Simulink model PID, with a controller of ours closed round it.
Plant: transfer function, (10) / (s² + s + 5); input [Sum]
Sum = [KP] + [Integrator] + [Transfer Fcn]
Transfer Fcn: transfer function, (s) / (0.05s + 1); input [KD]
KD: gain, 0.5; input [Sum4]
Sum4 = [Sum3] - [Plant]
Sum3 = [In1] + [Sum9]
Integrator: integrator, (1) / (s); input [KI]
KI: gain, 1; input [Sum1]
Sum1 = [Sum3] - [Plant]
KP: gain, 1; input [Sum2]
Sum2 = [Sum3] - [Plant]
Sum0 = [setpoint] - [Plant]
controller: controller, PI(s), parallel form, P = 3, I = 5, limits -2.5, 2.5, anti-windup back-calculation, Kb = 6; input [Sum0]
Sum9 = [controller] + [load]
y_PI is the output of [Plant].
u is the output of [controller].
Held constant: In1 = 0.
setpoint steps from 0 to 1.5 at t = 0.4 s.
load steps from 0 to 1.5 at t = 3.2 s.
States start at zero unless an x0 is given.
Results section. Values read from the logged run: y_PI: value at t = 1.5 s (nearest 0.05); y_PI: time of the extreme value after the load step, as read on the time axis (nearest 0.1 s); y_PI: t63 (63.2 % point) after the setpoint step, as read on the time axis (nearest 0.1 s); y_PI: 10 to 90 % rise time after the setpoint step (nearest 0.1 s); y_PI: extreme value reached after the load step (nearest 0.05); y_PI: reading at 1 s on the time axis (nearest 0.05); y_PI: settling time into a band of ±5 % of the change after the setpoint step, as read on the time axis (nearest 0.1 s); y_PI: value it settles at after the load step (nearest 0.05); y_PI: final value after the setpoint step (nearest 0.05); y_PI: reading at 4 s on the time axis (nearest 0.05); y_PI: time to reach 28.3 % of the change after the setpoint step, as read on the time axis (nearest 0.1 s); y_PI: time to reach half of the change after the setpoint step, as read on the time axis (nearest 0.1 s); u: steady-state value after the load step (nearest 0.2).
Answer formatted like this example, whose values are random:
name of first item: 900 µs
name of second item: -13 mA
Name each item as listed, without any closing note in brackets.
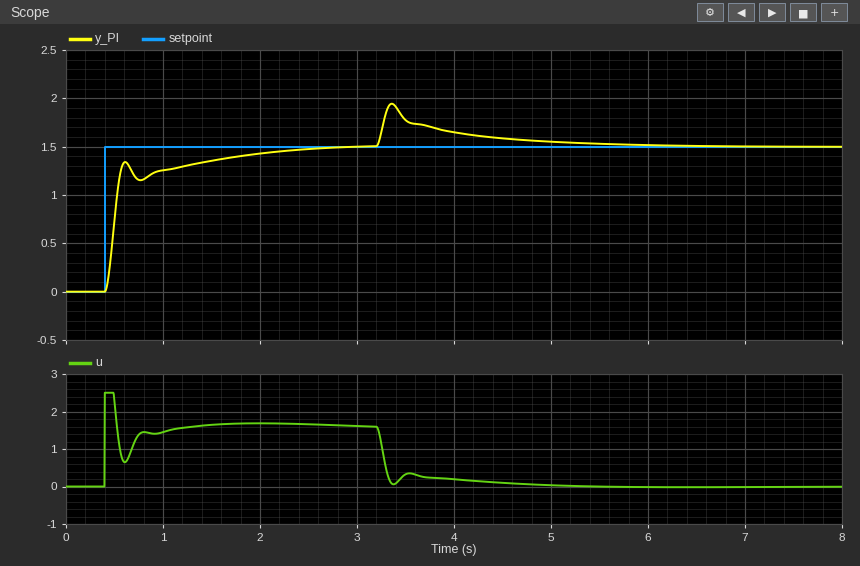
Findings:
y_PI: value at t = 1.5 s: 1.35
y_PI: time of the extreme value after the load step, as read on the time axis: 3.4 s
y_PI: t63 (63.2 % point) after the setpoint step, as read on the time axis: 0.5 s
y_PI: 10 to 90 % rise time after the setpoint step: 1.0 s
y_PI: extreme value reached after the load step: 1.95
y_PI: reading at 1 s on the time axis: 1.25
y_PI: settling time into a band of ±5 % of the change after the setpoint step, as read on the time axis: 2.0 s
y_PI: value it settles at after the load step: 1.50
y_PI: final value after the setpoint step: 1.50
y_PI: reading at 4 s on the time axis: 1.65
y_PI: time to reach 28.3 % of the change after the setpoint step, as read on the time axis: 0.5 s
y_PI: time to reach half of the change after the setpoint step, as read on the time axis: 0.5 s
u: steady-state value after the load step: 0.0
